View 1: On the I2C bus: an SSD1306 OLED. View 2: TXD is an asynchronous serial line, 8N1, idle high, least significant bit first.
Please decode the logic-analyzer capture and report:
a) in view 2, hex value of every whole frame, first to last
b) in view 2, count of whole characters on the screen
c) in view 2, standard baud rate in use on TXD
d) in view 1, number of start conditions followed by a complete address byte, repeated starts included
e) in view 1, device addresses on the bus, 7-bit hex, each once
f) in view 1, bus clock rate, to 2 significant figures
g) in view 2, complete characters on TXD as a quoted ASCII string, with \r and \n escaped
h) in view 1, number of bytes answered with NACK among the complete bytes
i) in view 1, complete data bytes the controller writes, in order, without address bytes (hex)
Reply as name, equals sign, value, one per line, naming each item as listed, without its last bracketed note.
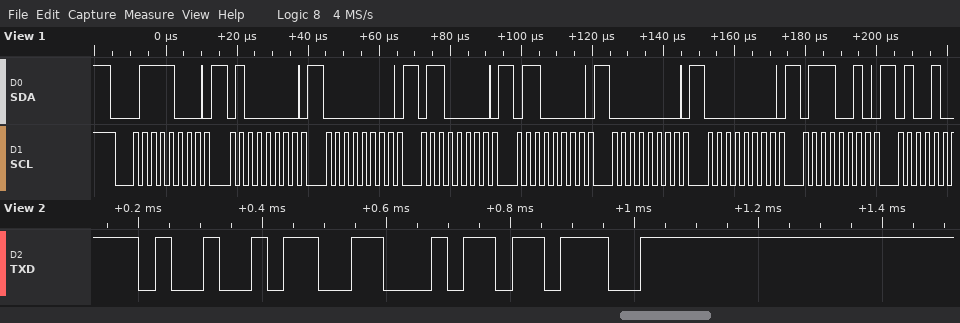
in view 2, hex value of every whole frame, first to last = 49 46 3B
in view 2, count of whole characters on the screen = 3
in view 2, standard baud rate in use on TXD = 38400 baud
in view 1, number of start conditions followed by a complete address byte, repeated starts included = 1
in view 1, device addresses on the bus, 7-bit hex, each once = 0x3C
in view 1, bus clock rate, to 2 significant figures = 400 kHz
in view 2, complete characters on TXD as a quoted ASCII string, with \r and \n escaped = "IF;"
in view 1, number of bytes answered with NACK among the complete bytes = 0
in view 1, complete data bytes the controller writes, in order, without address bytes = 40 00 60 60 00 00 72
